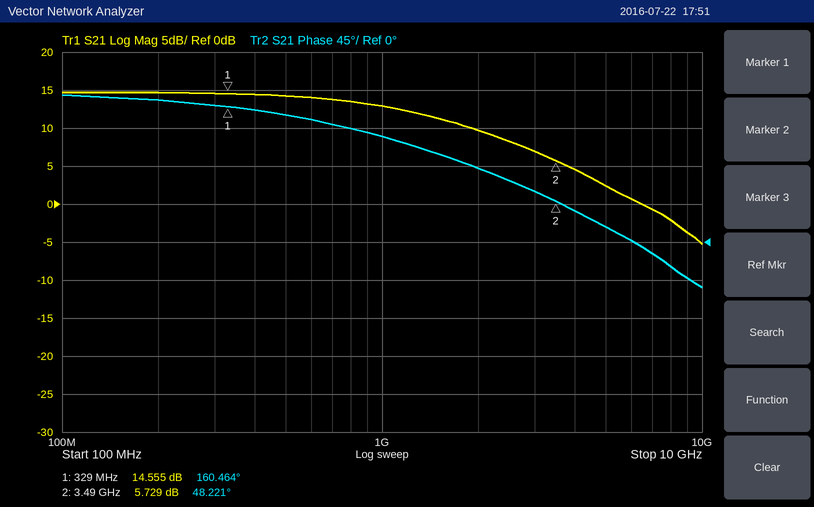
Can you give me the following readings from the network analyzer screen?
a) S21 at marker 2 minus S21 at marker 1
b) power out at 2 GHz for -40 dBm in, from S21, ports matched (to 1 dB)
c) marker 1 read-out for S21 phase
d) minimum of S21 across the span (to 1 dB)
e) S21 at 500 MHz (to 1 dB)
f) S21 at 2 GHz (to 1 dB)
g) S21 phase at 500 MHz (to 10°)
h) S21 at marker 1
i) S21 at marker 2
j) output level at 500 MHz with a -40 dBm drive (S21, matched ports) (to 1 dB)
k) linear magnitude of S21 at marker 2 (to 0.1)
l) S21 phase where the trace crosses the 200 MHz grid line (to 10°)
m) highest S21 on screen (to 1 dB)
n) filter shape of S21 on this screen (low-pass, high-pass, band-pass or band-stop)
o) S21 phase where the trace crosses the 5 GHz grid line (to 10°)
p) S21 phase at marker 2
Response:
-8.826 dB
-30 dBm
160.464°
-5 dB
14 dB
10 dB
150°
14.555 dB
5.729 dB
-26 dBm
1.9
170°
15 dB
low-pass
20°
48.221°
